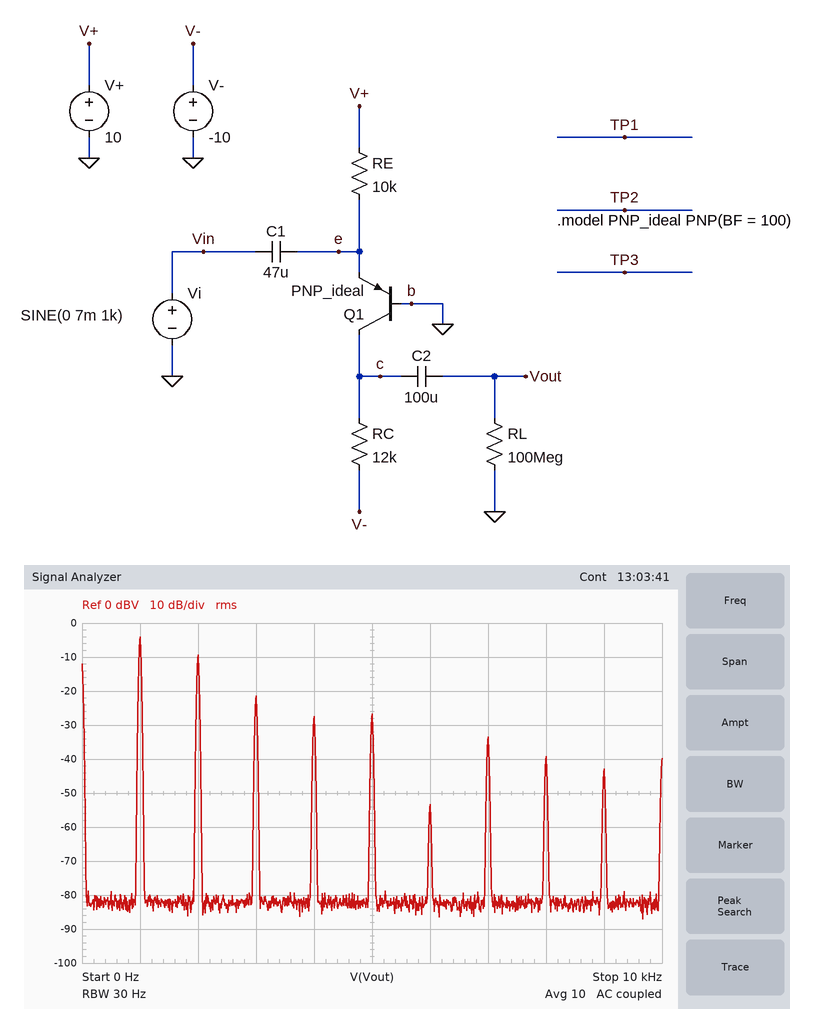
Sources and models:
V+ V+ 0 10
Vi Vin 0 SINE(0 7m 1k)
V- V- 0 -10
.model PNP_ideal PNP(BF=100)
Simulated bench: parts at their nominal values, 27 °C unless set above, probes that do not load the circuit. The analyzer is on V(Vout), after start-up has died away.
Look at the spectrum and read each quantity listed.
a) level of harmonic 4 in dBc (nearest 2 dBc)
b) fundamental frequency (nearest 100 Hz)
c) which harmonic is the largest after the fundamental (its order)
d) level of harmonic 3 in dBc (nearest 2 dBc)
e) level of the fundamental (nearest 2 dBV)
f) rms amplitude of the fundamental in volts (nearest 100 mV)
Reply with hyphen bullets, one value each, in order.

- -24 dBc
- 1.0 kHz
- 2
- -18 dBc
- -4 dBV
- 600 mV
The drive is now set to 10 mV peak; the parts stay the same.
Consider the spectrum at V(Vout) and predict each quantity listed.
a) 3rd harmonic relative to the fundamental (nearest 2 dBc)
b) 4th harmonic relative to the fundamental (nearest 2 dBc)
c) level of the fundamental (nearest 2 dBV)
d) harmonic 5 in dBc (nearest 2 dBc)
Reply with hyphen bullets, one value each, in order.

- -22 dBc
- -20 dBc
- 0 dBV
- -24 dBc
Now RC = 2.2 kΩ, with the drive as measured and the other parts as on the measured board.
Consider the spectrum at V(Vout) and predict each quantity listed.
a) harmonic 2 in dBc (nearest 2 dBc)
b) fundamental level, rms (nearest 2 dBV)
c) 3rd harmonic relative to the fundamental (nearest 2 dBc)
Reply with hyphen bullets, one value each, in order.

- -24 dBc
- -8 dBV
- -50 dBc
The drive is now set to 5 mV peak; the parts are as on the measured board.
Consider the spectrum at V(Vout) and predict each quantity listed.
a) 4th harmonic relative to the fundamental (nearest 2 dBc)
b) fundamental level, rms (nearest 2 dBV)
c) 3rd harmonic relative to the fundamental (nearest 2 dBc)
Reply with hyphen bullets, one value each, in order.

- -30 dBc
- -8 dBV
- -14 dBc
